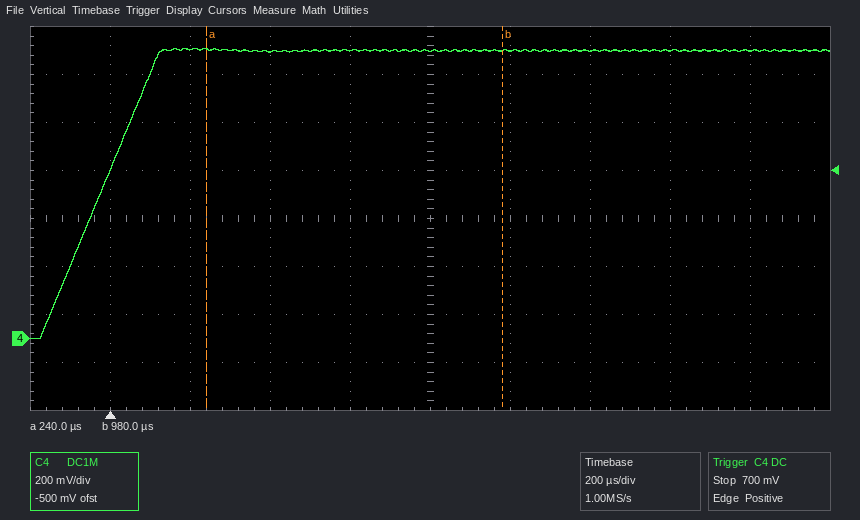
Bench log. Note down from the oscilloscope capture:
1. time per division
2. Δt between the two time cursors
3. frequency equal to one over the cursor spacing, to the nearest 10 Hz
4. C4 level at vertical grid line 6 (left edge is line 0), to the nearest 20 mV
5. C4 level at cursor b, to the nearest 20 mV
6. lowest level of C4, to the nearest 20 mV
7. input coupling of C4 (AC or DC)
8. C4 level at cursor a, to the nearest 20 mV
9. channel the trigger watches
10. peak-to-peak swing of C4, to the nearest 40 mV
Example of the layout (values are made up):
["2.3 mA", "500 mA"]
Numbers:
["200 µs", "740 µs", "1.35 kHz", "1.20 V", "1.20 V", "0 mV", "DC", "1.20 V", "C4", "1.20 V"]
